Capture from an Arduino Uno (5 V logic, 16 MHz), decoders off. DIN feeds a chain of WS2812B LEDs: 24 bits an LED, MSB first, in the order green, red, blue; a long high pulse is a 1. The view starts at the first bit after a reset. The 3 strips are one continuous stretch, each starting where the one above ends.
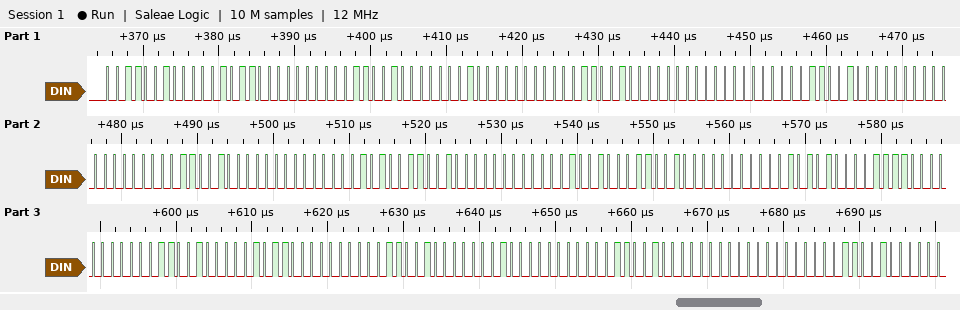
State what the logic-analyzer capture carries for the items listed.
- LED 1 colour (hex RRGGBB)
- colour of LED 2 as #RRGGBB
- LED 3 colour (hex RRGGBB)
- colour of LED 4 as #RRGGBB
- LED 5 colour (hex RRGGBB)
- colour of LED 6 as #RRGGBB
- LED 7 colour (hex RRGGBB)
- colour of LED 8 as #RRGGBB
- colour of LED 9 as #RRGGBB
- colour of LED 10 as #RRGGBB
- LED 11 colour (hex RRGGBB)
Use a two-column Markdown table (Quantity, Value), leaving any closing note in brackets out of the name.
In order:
| Quantity | Value |
|---|---|
| LED 1 colour | #0B3200 |
| colour of LED 2 as #RRGGBB | #023200 |
| LED 3 colour | #003200 |
| colour of LED 4 as #RRGGBB | #003200 |
| LED 5 colour | #003205 |
| colour of LED 6 as #RRGGBB | #003212 |
| LED 7 colour | #00322A |
| colour of LED 8 as #RRGGBB | #001E32 |
| colour of LED 9 as #RRGGBB | #000B32 |
| colour of LED 10 as #RRGGBB | #000232 |
| LED 11 colour | #000032 |
